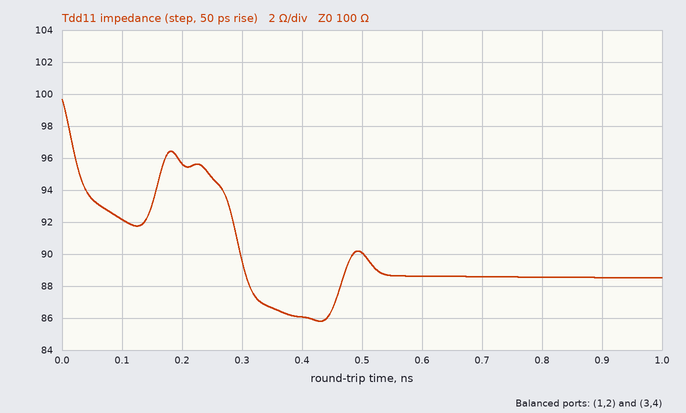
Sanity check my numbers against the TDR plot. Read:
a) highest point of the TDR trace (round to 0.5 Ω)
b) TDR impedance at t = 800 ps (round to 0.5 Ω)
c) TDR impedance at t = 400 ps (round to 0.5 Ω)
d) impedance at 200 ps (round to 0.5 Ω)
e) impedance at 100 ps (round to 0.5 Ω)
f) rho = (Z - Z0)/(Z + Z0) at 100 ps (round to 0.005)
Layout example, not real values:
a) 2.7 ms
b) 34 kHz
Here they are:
a) 99.5 Ω
b) 88.5 Ω
c) 86.0 Ω
d) 95.5 Ω
e) 92.0 Ω
f) -0.040
